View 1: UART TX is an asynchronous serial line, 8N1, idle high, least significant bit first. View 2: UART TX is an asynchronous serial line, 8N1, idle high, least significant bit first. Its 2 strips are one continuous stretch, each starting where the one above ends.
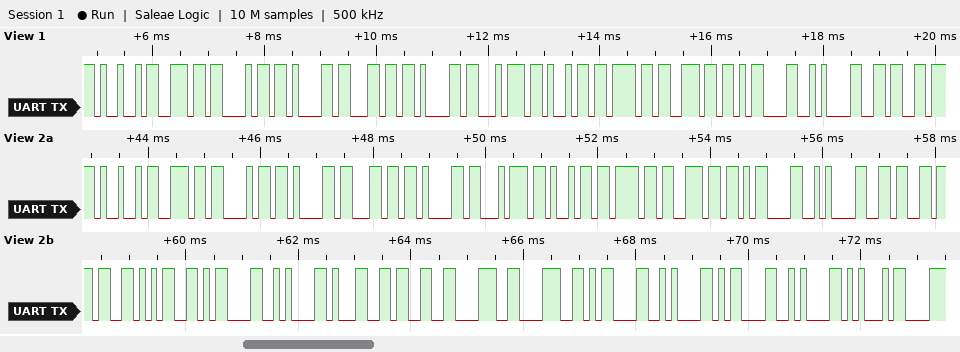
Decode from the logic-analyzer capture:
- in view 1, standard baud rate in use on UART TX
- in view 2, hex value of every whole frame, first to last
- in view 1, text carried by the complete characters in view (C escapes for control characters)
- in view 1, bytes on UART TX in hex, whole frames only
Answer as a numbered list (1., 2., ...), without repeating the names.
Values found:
1. 9600 baud
2. 49 6E 68 61 6C 61 74 69 6F 6E 0D 0A 36 37 35 0D 0A 31 33 38 38 0D 0A 0D 0A 45
3. "Inhalation\r\n6"
4. 49 6E 68 61 6C 61 74 69 6F 6E 0D 0A 36
